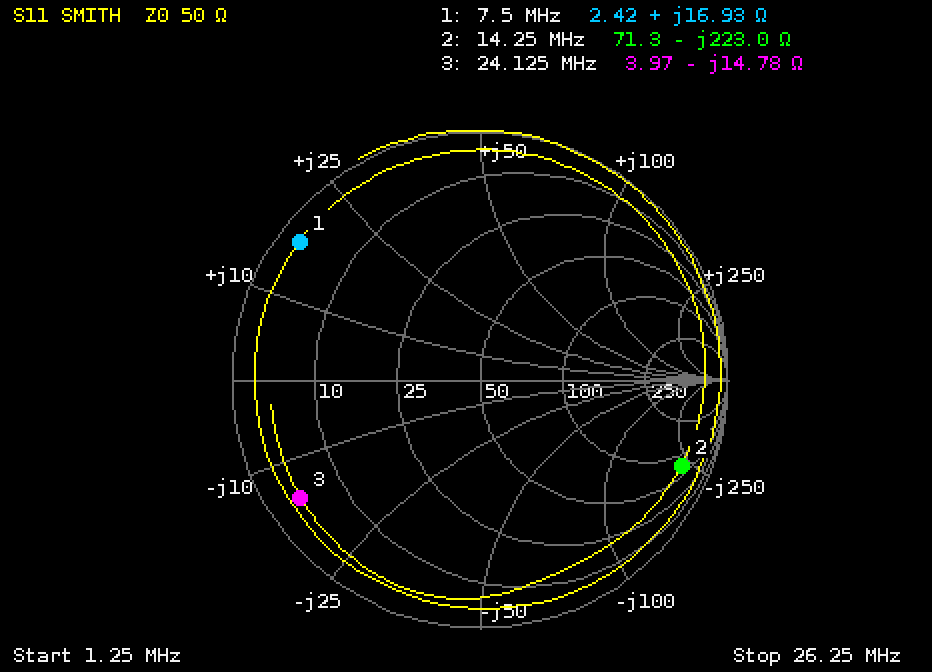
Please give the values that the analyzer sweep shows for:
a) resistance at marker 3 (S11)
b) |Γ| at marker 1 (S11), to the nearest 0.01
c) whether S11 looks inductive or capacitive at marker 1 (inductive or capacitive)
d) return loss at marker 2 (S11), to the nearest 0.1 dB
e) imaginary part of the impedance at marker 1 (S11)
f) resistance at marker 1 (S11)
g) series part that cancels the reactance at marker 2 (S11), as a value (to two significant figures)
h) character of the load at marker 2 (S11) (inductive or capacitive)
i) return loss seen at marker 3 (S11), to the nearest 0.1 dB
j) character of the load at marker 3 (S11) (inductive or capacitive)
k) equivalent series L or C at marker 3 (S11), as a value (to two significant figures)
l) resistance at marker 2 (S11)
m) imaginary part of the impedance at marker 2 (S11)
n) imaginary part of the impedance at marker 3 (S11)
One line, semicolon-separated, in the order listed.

3.97 Ω; 0.92; inductive; 1.1 dB; +16.93 Ω; 2.42 Ω; 2.5 µH; capacitive; 1.3 dB; capacitive; 450 pF; 71.3 Ω; -223.0 Ω; -14.78 Ω
